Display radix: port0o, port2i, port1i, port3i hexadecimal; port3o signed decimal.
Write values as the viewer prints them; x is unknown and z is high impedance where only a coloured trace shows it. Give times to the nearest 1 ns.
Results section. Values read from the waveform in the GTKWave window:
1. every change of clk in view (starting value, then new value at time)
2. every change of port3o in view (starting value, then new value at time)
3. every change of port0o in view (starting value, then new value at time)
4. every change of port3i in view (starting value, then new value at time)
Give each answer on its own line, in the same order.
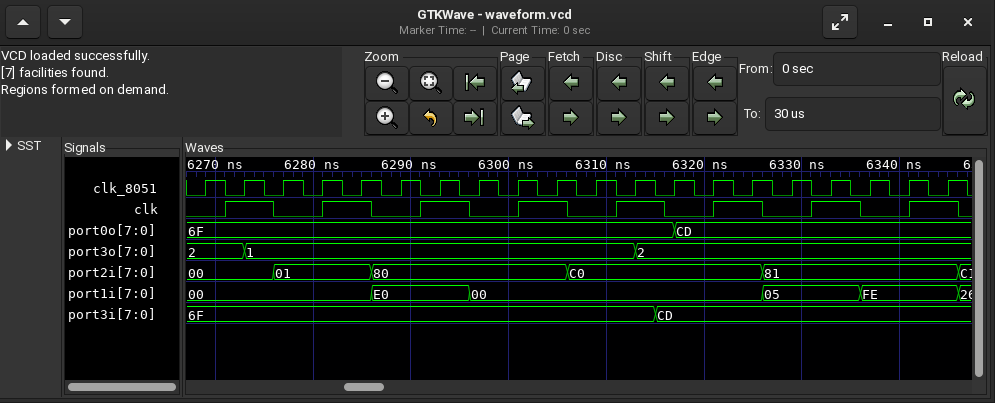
0, 1 at 6271 ns, 0 at 6276 ns, 1 at 6281 ns, 0 at 6286 ns, 1 at 6291 ns, 0 at 6296 ns, 1 at 6301 ns, 0 at 6306 ns, 1 at 6311 ns, 0 at 6316 ns, 1 at 6321 ns, 0 at 6326 ns, 1 at 6331 ns, 0 at 6336 ns, 1 at 6341 ns, 0 at 6346 ns
2, 1 at 6273 ns, 2 at 6313 ns
6F, CD at 6317 ns
6F, CD at 6315 ns
